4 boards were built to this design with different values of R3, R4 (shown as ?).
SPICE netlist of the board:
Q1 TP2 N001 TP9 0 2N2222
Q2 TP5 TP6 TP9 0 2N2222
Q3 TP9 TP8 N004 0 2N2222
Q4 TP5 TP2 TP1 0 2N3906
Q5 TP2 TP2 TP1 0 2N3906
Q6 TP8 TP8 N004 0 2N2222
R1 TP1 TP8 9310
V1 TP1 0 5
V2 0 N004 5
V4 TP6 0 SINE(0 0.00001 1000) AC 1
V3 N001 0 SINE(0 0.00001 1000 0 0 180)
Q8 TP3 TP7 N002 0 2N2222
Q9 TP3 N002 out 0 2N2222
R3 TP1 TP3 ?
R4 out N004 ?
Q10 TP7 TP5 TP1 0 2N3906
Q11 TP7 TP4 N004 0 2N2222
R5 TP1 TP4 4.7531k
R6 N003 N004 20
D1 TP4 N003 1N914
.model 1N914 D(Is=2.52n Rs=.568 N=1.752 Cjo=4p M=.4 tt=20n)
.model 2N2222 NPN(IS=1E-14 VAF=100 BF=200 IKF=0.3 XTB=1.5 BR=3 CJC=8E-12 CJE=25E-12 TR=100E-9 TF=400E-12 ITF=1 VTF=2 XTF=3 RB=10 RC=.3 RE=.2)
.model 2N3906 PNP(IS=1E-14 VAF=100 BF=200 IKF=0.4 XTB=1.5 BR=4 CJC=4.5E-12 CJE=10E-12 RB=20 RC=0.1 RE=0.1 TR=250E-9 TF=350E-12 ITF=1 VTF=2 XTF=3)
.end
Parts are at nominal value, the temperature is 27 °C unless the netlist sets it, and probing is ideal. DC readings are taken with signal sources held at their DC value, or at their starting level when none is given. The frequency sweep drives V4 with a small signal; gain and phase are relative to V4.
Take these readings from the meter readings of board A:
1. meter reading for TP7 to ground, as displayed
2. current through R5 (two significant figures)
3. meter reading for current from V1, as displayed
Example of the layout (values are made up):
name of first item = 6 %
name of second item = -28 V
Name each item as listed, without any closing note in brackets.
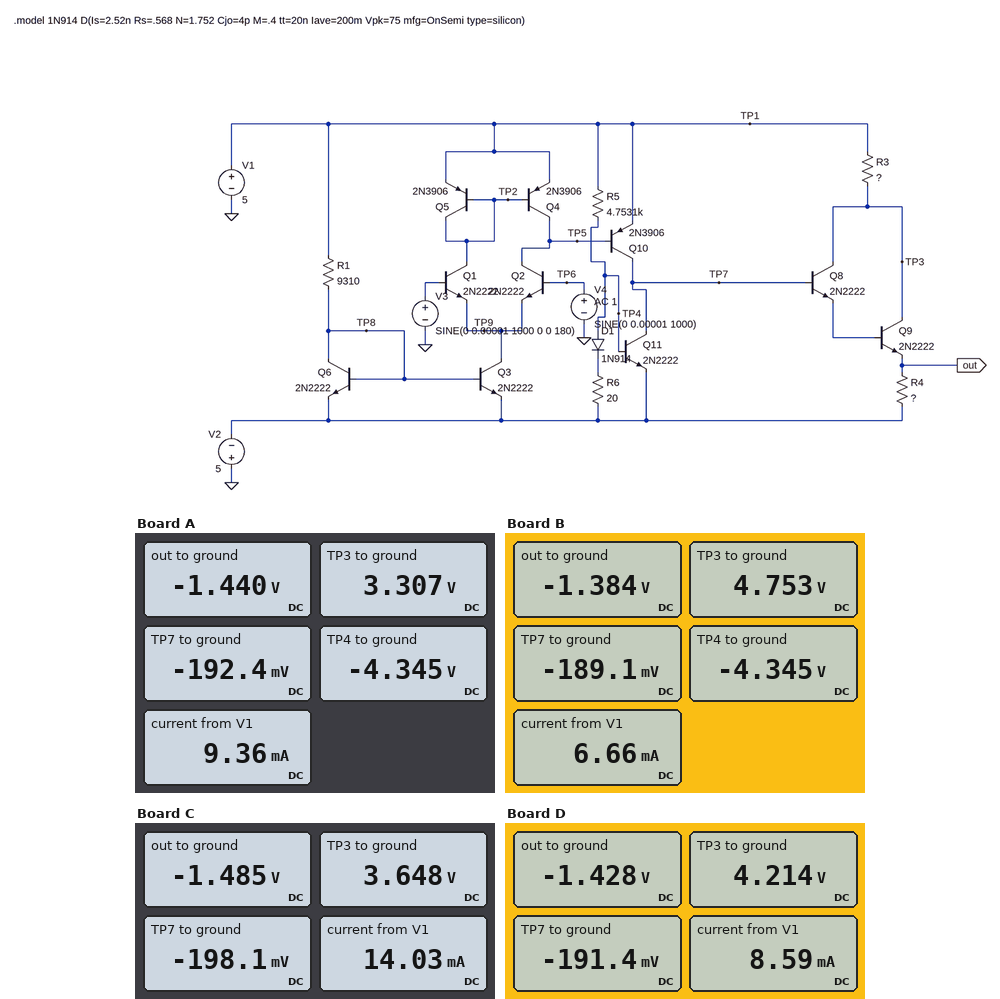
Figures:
meter reading for TP7 to ground, as displayed = -192.4 mV
current through R5 = 2.0 mA
meter reading for current from V1, as displayed = 9.36 mA
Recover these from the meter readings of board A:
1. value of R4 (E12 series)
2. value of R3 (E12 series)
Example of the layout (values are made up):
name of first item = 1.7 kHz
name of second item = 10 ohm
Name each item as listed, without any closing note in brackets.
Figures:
value of R4 = 820 Ω
value of R3 = 390 Ω
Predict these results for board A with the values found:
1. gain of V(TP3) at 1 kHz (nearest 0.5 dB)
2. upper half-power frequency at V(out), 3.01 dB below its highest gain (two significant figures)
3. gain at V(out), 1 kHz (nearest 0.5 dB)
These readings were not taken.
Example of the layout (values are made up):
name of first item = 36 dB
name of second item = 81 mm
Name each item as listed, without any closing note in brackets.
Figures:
gain of V(TP3) at 1 kHz = 99.0 dB
upper half-power frequency at V(out), 3.01 dB below its highest gain = 6.3 kHz
gain at V(out), 1 kHz = 105.5 dB
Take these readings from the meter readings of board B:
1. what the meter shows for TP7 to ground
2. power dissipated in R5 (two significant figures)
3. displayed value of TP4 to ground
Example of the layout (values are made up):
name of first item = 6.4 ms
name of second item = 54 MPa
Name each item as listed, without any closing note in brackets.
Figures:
what the meter shows for TP7 to ground = -189.1 mV
power dissipated in R5 = 18 mW
displayed value of TP4 to ground = -4.345 V
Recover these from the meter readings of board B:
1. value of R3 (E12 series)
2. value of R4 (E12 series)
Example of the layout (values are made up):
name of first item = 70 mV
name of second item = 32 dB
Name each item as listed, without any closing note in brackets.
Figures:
value of R3 = 150 Ω
value of R4 = 2.2 kΩ
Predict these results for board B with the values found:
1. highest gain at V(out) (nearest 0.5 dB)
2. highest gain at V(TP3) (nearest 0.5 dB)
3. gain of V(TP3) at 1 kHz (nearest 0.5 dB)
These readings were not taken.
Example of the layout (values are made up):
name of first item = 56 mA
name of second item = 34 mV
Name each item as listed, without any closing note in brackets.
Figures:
highest gain at V(out) = 106.0 dB
highest gain at V(TP3) = 82.5 dB
gain of V(TP3) at 1 kHz = 82.5 dB
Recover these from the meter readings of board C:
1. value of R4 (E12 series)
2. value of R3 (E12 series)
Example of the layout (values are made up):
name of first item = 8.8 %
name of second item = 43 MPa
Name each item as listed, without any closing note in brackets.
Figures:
value of R4 = 390 Ω
value of R3 = 150 Ω
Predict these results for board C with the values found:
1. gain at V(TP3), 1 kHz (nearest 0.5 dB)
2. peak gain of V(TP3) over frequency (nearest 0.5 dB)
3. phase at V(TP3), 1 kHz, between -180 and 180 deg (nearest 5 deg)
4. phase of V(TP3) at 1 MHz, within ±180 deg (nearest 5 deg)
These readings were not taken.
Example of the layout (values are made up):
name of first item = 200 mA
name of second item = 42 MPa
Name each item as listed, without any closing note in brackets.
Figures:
gain at V(TP3), 1 kHz = 97.5 dB
peak gain of V(TP3) over frequency = 97.5 dB
phase at V(TP3), 1 kHz, between -180 and 180 deg = 170 deg
phase of V(TP3) at 1 MHz, within ±180 deg = 85 deg
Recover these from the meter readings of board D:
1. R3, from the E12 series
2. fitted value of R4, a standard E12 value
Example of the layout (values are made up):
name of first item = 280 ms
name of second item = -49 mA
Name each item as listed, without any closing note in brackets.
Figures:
R3, from the E12 series = 220 Ω
fitted value of R4, a standard E12 value = 1 kΩ
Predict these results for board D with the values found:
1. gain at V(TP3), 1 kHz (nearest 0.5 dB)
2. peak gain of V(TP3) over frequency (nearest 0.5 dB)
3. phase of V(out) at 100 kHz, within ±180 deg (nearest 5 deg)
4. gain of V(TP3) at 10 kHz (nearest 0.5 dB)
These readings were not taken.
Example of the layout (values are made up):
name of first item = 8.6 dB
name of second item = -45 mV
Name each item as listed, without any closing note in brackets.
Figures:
gain at V(TP3), 1 kHz = 92.5 dB
peak gain of V(TP3) over frequency = 92.5 dB
phase of V(out) at 100 kHz, within ±180 deg = -85 deg
gain of V(TP3) at 10 kHz = 87.0 dB
